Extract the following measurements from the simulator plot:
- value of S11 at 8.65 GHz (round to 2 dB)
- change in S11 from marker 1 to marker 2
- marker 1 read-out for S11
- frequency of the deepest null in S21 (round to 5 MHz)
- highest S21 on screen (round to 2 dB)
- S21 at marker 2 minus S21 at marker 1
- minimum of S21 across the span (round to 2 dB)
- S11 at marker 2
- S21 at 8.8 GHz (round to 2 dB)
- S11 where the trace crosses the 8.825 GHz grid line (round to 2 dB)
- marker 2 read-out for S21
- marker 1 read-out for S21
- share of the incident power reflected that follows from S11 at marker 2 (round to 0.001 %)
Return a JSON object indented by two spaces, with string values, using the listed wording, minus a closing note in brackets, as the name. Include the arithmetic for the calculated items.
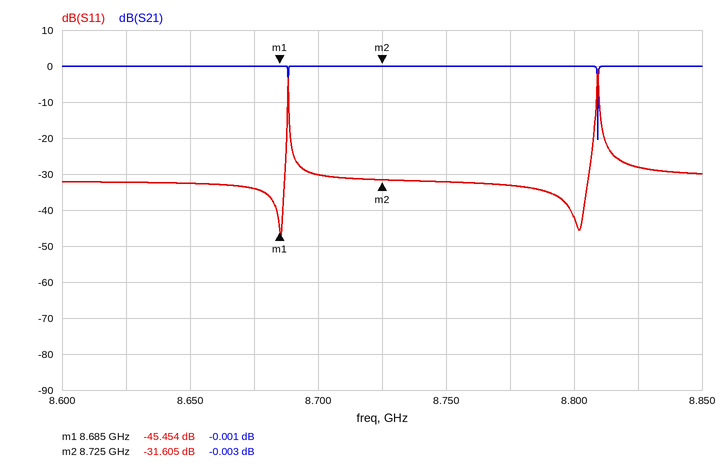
{
  "value of S11 at 8.65 GHz": "-32 dB",
  "change in S11 from marker 1 to marker 2": "-31.605 − (-45.454) = 13.849 dB",
  "marker 1 read-out for S11": "-45.454 dB",
  "frequency of the deepest null in S21": "8.810 GHz",
  "highest S21 on screen": "0 dB",
  "S21 at marker 2 minus S21 at marker 1": "-0.003 − (-0.001) = -0.002 dB",
  "minimum of S21 across the span": "-20 dB",
  "S11 at marker 2": "-31.605 dB",
  "S21 at 8.8 GHz": "0 dB",
  "S11 where the trace crosses the 8.825 GHz grid line": "-28 dB",
  "marker 2 read-out for S21": "-0.003 dB",
  "marker 1 read-out for S21": "-0.001 dB",
  "share of the incident power reflected that follows from S11 at marker 2": "10^(-31.605/10) ≈ 0.069 %"
}
